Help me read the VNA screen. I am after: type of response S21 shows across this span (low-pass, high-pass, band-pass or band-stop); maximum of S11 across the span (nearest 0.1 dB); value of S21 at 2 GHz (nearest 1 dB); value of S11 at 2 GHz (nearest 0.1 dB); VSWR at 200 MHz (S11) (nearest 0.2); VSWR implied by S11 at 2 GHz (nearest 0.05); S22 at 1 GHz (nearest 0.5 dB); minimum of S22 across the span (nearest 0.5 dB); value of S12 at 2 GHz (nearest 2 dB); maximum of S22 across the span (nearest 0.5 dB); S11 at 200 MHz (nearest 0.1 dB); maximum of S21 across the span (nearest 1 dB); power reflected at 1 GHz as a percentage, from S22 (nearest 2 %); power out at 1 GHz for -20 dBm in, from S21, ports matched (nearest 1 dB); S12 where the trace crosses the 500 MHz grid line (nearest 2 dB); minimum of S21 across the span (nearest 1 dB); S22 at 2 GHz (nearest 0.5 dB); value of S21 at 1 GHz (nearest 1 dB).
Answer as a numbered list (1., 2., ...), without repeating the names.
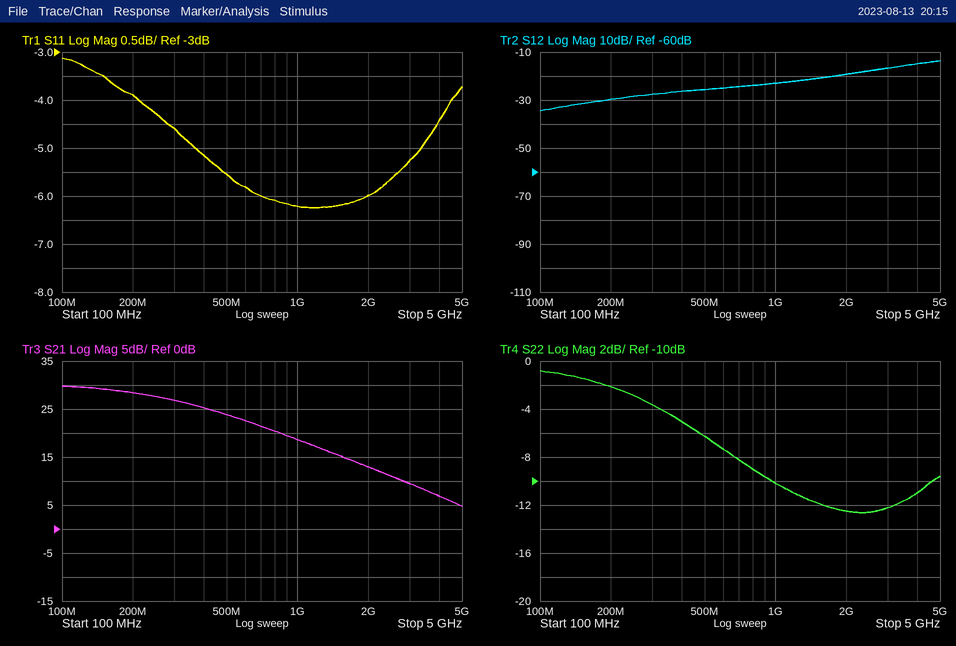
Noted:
1. low-pass
2. -3.1 dB
3. 13 dB
4. -6.0 dB
5. 4.6
6. 3.00
7. -10.0 dB
8. -12.5 dB
9. -20 dB
10. -1.0 dB
11. -3.9 dB
12. 30 dB
13. 10 %
14. -1 dBm
15. -26 dB
16. 5 dB
17. -12.5 dB
18. 19 dB
